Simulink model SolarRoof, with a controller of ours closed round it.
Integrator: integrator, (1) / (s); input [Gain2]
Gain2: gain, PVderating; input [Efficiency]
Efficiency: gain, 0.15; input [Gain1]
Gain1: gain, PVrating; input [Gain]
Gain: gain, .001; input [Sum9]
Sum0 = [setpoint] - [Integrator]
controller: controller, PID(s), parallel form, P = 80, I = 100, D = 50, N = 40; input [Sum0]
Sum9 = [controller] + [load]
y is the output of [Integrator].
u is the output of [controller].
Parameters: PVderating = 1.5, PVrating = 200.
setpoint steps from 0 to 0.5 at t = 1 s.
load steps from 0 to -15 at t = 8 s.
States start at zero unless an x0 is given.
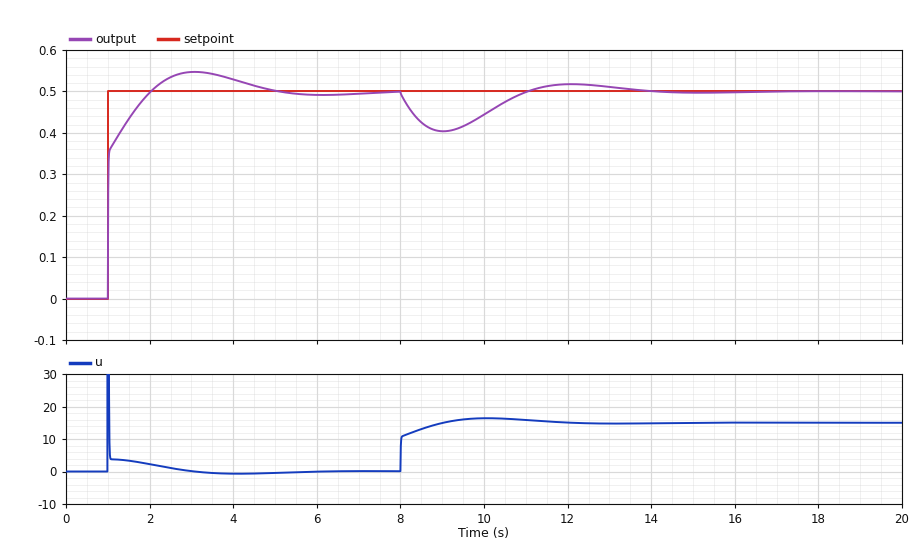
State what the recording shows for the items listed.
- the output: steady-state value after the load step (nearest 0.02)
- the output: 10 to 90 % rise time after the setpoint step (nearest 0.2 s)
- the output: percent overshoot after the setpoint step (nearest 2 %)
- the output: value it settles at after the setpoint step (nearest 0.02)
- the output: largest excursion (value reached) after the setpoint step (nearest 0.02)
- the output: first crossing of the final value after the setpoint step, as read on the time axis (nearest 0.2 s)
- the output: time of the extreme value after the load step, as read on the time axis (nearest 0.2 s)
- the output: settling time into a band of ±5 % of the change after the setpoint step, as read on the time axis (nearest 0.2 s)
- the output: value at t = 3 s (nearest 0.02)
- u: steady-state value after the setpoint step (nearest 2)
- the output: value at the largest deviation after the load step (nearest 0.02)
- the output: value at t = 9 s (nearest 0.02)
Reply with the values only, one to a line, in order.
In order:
0.50
0.6 s
10 %
0.50
0.54
2.0 s
9.0 s
4.2 s
0.54
0
0.40
0.40
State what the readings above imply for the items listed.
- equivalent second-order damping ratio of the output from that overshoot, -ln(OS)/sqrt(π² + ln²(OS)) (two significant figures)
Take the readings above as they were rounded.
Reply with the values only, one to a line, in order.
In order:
0.59
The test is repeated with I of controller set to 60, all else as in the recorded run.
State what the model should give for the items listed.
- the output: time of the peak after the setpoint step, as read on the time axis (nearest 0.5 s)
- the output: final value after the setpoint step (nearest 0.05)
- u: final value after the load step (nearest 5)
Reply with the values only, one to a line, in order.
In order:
3.5 s
0.50
15
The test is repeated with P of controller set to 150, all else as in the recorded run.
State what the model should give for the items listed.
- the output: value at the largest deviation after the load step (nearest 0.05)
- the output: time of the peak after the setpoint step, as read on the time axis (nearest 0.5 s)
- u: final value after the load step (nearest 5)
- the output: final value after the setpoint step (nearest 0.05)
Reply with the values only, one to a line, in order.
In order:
0.45
3.0 s
15
0.50
